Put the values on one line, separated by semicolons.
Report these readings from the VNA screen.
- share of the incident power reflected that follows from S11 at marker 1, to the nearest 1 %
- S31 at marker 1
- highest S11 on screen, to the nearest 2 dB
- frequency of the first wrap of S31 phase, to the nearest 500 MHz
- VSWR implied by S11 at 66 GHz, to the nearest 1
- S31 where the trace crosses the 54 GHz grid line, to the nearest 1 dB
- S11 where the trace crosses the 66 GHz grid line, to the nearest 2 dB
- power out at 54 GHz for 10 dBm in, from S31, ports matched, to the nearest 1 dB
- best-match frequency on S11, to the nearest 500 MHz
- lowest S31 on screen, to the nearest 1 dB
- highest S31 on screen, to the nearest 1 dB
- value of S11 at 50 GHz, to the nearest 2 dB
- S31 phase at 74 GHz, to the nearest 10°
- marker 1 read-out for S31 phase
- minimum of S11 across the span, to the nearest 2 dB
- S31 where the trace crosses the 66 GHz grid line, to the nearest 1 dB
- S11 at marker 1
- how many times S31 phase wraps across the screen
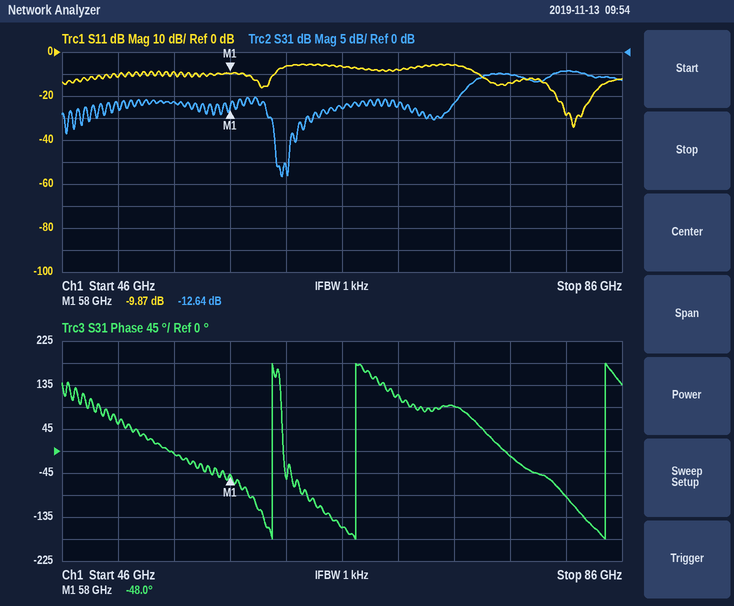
10 %; -12.64 dB; -6 dB; 61.0 GHz; 3; -11 dB; -6 dB; -1 dBm; 82.5 GHz; -28 dB; -4 dB; -12 dB; 90°; -48.0°; -34 dB; -13 dB; -9.87 dB; 3
